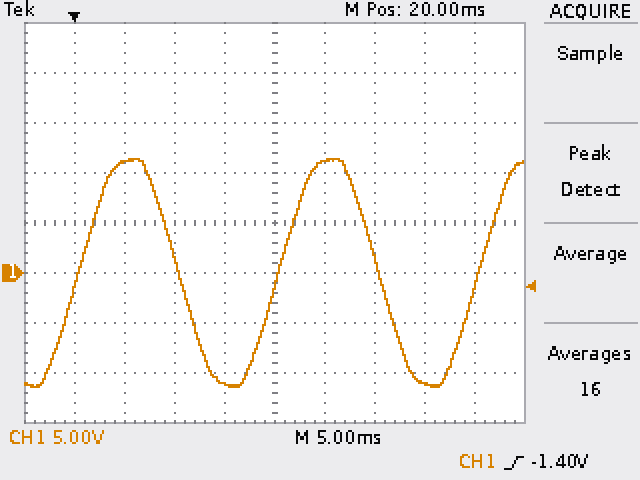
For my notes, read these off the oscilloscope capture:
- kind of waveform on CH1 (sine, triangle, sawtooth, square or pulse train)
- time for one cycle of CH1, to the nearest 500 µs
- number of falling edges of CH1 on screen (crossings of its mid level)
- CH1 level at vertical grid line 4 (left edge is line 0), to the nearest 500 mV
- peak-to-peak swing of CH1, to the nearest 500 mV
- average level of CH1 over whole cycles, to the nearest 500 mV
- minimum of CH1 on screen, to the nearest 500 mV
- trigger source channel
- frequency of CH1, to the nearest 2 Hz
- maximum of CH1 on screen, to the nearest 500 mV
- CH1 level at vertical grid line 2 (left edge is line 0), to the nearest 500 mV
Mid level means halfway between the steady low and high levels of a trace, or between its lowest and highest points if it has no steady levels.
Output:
sine
20.0 ms
2
-11.0 V
23.0 V
0.0 V
-11.5 V
CH1
50 Hz
11.5 V
11.0 V
